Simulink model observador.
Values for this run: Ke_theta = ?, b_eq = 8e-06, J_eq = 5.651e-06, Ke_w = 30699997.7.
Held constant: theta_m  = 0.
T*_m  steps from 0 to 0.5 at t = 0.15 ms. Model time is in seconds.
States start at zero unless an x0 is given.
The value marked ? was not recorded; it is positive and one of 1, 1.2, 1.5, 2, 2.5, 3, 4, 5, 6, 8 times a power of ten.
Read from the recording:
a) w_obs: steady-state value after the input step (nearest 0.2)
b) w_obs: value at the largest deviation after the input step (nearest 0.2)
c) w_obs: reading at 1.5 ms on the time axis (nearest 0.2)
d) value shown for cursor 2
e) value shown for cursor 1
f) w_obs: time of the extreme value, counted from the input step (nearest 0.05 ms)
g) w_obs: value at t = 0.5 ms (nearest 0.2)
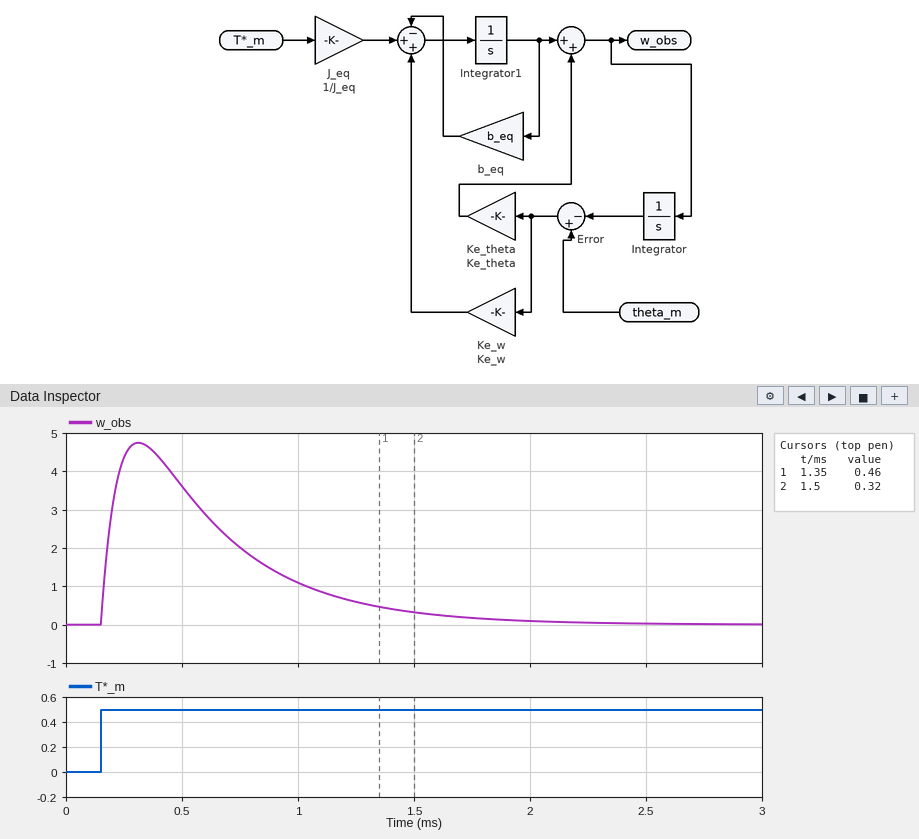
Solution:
0.0
4.8
0.4
0.32
0.46
0.15 ms
3.6
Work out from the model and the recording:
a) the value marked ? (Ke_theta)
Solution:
15000
